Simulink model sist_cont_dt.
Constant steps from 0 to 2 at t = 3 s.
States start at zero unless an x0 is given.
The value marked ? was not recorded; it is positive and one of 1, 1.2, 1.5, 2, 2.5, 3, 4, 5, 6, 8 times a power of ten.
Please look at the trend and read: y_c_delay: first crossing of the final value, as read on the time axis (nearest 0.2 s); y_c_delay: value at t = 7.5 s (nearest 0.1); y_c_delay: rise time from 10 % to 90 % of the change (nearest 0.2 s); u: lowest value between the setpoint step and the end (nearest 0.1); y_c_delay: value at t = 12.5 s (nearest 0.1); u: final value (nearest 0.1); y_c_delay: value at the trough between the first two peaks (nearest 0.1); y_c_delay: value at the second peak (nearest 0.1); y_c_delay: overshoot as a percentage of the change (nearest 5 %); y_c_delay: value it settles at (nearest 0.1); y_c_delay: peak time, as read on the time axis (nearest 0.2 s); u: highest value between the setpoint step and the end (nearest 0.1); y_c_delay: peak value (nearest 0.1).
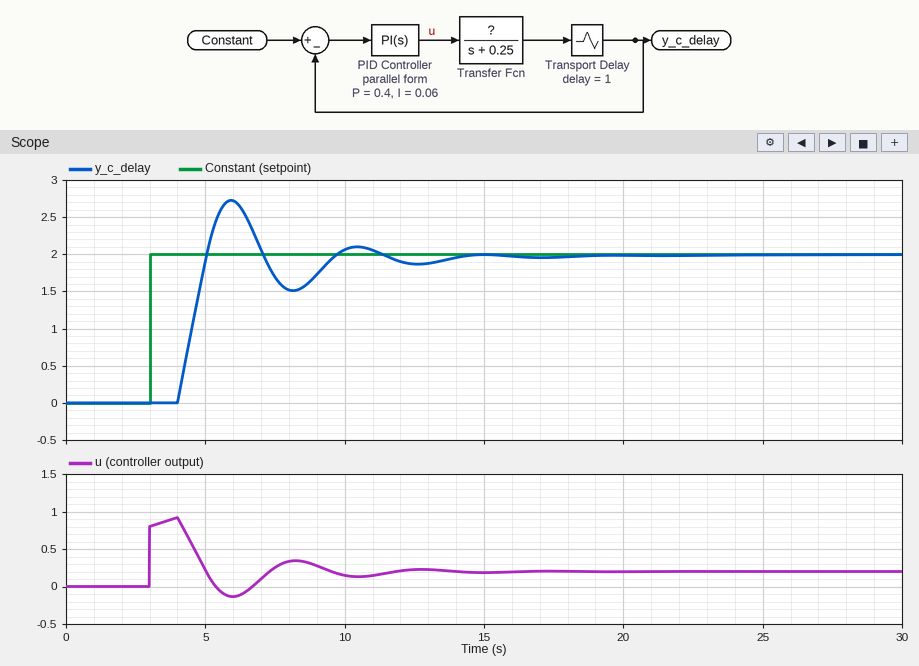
5.0 s
1.7
0.8 s
-0.1
1.9
0.2
1.5
2.1
35 %
2.0
6.0 s
0.9
2.7
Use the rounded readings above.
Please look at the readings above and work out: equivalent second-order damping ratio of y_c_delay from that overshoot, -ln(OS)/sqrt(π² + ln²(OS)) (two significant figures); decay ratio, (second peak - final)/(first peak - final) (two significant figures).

0.32
0.14
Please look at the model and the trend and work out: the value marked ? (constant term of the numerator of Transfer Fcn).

2.5
